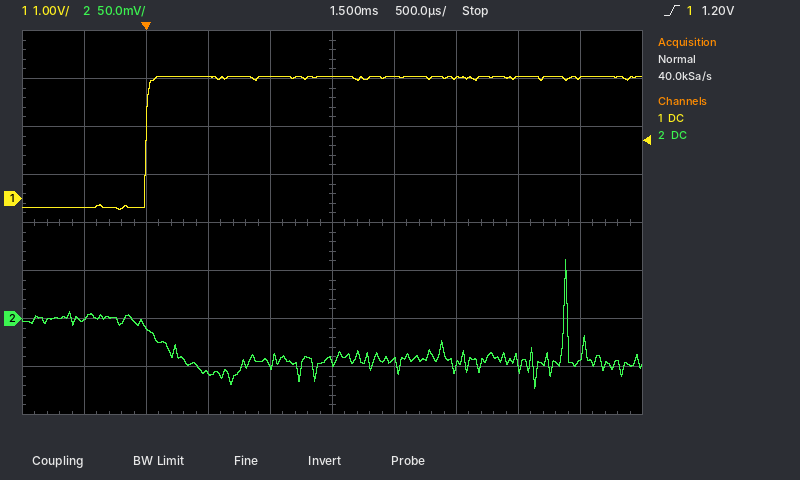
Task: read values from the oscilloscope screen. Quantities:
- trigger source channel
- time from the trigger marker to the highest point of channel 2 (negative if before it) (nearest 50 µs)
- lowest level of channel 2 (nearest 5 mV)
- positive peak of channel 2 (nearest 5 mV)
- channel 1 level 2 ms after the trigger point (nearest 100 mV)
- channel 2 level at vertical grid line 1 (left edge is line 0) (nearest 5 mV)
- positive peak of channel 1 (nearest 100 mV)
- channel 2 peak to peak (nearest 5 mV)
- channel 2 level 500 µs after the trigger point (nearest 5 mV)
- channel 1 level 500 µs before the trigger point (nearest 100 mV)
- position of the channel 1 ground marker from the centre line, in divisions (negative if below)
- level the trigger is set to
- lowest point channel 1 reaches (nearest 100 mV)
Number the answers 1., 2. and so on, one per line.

1. channel 1
2. +3.40 ms
3. -75 mV
4. 60 mV
5. 2.5 V
6. 0 mV
7. 2.5 V
8. 135 mV
9. -55 mV
10. -200 mV
11. +0.5 div
12. 1.20 V
13. -200 mV
